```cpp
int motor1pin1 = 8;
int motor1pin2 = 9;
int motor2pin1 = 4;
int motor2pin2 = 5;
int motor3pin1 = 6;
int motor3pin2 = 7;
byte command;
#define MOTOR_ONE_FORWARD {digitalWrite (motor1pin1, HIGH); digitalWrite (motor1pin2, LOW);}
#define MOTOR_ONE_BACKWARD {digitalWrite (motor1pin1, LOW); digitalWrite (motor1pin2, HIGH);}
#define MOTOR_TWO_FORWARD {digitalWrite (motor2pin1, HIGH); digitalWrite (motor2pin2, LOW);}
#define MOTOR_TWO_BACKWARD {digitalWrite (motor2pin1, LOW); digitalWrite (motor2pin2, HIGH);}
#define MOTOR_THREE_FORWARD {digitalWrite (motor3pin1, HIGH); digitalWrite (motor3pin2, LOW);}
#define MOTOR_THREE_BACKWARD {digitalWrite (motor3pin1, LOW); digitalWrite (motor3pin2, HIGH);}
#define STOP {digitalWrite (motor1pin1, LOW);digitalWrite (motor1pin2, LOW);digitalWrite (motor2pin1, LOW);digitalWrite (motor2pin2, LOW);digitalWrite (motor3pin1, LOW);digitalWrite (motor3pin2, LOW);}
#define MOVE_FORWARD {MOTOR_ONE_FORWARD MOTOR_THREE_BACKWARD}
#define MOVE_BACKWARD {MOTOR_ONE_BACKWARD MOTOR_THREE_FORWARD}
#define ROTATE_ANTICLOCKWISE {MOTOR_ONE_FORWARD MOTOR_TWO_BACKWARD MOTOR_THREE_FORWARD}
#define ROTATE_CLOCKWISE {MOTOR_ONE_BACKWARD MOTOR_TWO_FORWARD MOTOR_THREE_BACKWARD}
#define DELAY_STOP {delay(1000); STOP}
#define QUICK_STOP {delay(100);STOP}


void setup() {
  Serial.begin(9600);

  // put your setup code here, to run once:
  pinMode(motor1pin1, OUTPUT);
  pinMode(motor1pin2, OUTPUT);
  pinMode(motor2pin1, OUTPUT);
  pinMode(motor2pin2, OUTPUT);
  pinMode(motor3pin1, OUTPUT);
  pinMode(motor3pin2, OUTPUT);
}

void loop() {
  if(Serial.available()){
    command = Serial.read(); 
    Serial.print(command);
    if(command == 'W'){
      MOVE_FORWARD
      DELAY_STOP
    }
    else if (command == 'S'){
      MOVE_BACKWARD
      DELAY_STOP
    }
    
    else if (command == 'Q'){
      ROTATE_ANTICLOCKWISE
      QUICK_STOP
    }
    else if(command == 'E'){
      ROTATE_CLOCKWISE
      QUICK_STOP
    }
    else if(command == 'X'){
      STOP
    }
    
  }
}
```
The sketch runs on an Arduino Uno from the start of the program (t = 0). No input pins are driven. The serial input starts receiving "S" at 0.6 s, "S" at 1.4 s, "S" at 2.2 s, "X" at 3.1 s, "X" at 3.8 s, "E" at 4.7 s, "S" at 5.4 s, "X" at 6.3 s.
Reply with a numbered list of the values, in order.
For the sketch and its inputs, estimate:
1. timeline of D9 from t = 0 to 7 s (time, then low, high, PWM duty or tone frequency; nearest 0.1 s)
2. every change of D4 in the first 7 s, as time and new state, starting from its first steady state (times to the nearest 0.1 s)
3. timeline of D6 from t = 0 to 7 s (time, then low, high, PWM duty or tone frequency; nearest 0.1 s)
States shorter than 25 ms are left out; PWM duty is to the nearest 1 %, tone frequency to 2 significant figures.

1. 0 s low; 0.6 s high; 3.6 s low; 4.7 s high; 4.8 s low; 5.4 s high; 6.4 s low
2. 0 s low; 4.7 s high; 4.8 s low
3. 0 s low; 0.6 s high; 3.6 s low; 5.4 s high; 6.4 s low
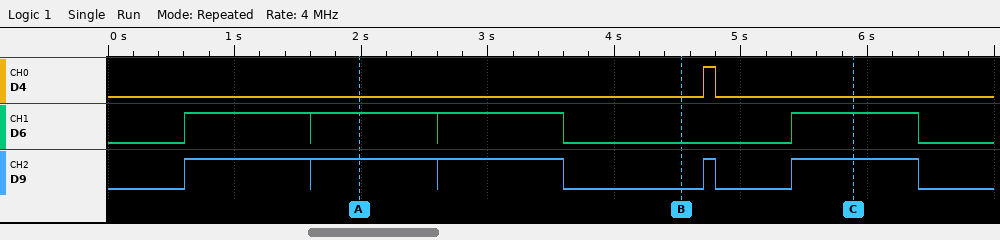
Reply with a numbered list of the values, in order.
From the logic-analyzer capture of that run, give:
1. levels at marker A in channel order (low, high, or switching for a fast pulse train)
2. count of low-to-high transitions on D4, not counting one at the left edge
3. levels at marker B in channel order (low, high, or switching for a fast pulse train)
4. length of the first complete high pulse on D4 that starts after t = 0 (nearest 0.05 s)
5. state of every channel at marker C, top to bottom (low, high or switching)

1. D4 low, D6 high, D9 high
2. 1
3. D4 low, D6 low, D9 low
4. 0.10 s
5. D4 low, D6 high, D9 high
